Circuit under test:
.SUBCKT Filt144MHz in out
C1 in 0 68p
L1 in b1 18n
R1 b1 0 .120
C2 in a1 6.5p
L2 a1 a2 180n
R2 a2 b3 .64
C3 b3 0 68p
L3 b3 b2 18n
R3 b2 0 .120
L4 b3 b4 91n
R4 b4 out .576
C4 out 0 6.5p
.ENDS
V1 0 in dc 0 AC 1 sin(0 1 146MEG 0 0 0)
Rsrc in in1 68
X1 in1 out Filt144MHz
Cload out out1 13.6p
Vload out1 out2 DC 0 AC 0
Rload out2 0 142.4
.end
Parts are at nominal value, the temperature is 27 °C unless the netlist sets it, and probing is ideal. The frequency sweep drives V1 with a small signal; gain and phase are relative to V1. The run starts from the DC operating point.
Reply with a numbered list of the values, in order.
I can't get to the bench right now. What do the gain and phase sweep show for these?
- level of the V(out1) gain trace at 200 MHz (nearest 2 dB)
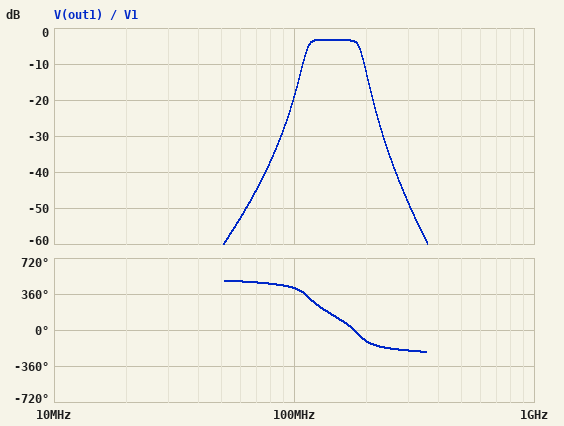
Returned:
1. -12 dB
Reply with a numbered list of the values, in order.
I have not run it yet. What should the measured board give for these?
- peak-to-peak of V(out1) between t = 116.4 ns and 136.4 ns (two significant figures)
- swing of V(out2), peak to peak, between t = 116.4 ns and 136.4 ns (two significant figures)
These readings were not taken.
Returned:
1. 1.4 V
2. 1.4 V
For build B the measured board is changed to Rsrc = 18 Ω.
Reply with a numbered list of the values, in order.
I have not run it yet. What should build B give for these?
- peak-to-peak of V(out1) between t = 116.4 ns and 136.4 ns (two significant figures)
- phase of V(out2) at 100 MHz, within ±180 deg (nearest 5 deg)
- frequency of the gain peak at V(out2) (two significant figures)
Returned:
1. 2.4 V
2. 25 deg
3. 160 MHz
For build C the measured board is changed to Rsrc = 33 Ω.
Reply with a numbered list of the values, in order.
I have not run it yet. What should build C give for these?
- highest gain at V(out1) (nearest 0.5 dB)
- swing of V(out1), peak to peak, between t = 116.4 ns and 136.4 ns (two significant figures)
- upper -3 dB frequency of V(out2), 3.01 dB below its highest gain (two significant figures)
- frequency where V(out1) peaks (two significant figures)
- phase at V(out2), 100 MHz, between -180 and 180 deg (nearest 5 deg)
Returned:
1. 0 dB
2. 2.0 V
3. 190 MHz
4. 150 MHz
5. 45 deg
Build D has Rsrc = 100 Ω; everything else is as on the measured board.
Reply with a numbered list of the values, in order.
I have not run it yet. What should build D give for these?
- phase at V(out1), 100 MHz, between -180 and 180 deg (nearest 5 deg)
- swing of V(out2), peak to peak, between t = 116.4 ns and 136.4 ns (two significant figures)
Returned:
1. 65 deg
2. 1.1 V
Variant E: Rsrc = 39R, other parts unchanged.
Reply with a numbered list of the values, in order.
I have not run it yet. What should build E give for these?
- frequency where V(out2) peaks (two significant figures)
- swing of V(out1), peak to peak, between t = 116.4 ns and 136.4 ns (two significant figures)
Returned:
1. 150 MHz
2. 1.8 V
